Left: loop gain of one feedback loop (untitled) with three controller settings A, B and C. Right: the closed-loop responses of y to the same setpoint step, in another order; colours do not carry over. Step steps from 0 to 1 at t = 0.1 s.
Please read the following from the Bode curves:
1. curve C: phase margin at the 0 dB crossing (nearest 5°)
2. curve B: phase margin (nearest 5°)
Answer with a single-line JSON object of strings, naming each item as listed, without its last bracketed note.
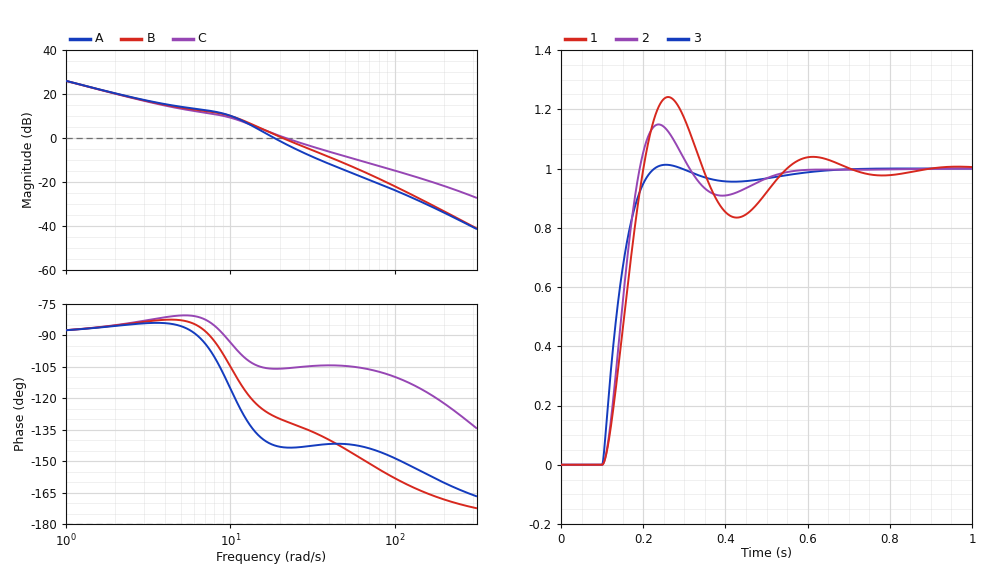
{"curve C: phase margin at the 0 dB crossing": "75°", "curve B: phase margin": "50°"}
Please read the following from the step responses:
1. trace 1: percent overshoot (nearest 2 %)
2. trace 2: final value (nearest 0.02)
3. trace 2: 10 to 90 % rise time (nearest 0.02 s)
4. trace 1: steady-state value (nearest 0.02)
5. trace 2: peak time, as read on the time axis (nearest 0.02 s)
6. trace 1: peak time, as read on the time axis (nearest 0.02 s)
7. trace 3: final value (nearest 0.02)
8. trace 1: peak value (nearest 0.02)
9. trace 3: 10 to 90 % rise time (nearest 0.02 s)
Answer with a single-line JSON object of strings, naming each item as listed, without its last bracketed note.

{"trace 1: percent overshoot": "24 %", "trace 2: final value": "1.00", "trace 2: 10 to 90 % rise time": "0.06 s", "trace 1: steady-state value": "1.00", "trace 2: peak time, as read on the time axis": "0.24 s", "trace 1: peak time, as read on the time axis": "0.26 s", "trace 3: final value": "1.00", "trace 1: peak value": "1.24", "trace 3: 10 to 90 % rise time": "0.08 s"}
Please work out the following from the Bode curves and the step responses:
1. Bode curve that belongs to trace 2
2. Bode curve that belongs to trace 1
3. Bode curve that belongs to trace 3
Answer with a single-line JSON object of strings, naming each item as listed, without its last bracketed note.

{"Bode curve that belongs to trace 2": "B", "Bode curve that belongs to trace 1": "A", "Bode curve that belongs to trace 3": "C"}
